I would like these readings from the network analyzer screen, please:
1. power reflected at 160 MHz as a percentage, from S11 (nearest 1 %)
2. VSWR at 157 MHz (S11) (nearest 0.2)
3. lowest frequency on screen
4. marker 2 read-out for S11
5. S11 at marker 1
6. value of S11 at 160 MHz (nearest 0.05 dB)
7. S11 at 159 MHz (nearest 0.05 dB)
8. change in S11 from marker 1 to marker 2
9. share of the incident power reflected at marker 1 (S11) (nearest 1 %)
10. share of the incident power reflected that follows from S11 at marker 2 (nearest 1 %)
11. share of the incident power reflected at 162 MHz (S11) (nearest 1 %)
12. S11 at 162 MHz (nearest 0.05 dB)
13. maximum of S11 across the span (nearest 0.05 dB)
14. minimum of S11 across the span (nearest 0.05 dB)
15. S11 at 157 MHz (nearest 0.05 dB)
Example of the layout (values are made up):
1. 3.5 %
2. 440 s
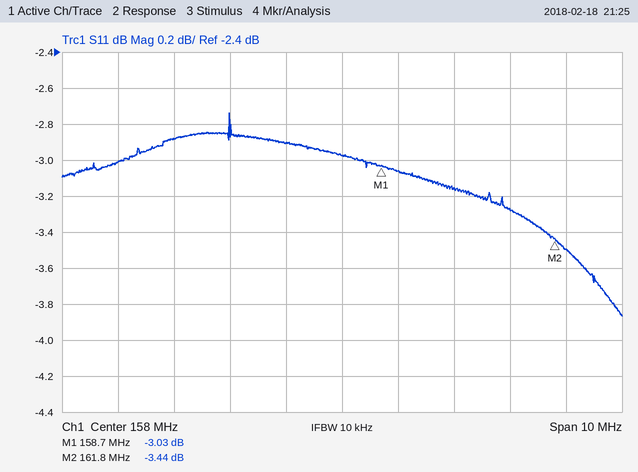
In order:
1. 48 %
2. 6.0
3. 153 MHz
4. -3.44 dB
5. -3.03 dB
6. -3.15 dB
7. -3.05 dB
8. -0.41 dB
9. 50 %
10. 45 %
11. 45 %
12. -3.50 dB
13. -2.75 dB
14. -3.85 dB
15. -2.90 dB
